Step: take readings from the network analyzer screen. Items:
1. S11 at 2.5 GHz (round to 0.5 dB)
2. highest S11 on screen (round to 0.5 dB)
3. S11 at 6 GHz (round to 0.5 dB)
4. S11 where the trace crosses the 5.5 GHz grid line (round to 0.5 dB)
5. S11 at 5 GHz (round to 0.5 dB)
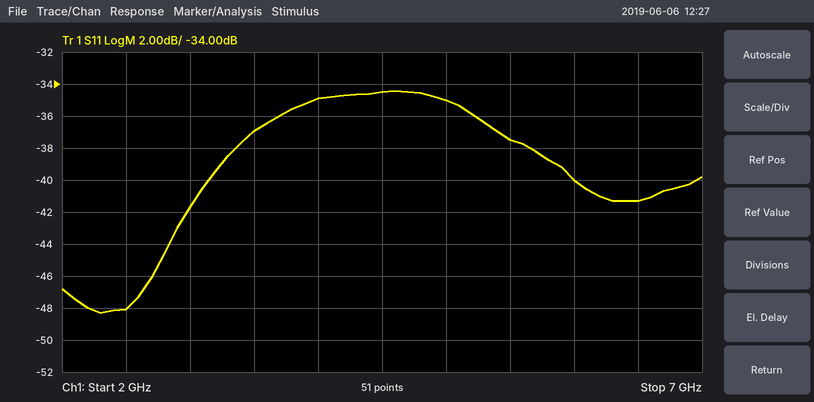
-48.0 dB
-34.5 dB
-40.0 dB
-37.5 dB
-35.0 dB
